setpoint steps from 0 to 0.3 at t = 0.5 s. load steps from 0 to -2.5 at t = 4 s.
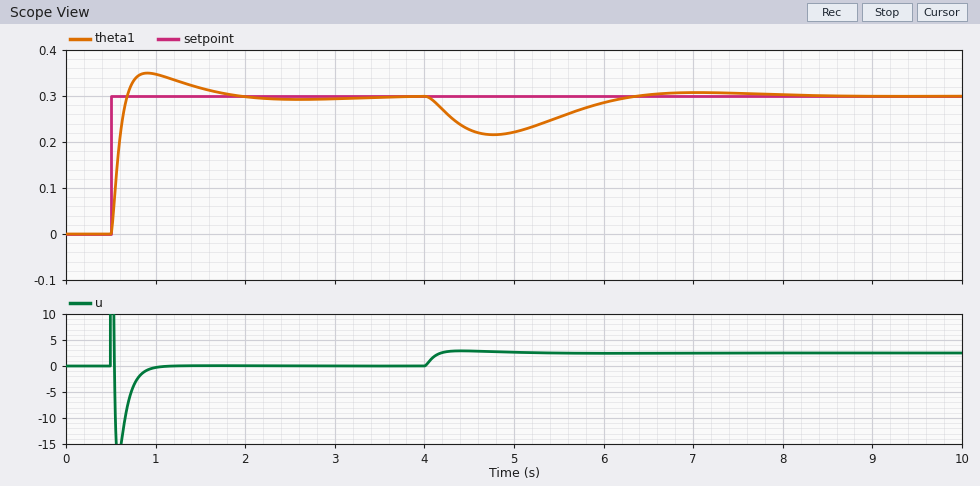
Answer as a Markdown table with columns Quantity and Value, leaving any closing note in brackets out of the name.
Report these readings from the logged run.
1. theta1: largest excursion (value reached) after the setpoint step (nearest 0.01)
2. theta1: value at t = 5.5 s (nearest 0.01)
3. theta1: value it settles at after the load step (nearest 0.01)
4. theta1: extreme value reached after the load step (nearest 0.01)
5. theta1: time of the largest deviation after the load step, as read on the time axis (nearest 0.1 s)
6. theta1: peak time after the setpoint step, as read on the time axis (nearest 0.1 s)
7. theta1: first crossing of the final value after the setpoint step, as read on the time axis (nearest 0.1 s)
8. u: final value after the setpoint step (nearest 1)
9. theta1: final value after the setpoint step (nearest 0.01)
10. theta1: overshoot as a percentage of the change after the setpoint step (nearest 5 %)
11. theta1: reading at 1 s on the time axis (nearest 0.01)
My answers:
| Quantity | Value |
|---|---|
| theta1: largest excursion (value reached) after the setpoint step | 0.35 |
| theta1: value at t = 5.5 s | 0.25 |
| theta1: value it settles at after the load step | 0.30 |
| theta1: extreme value reached after the load step | 0.22 |
| theta1: time of the largest deviation after the load step, as read on the time axis | 4.8 s |
| theta1: peak time after the setpoint step, as read on the time axis | 0.9 s |
| theta1: first crossing of the final value after the setpoint step, as read on the time axis | 0.7 s |
| u: final value after the setpoint step | 0 |
| theta1: final value after the setpoint step | 0.30 |
| theta1: overshoot as a percentage of the change after the setpoint step | 15 % |
| theta1: reading at 1 s on the time axis | 0.35 |
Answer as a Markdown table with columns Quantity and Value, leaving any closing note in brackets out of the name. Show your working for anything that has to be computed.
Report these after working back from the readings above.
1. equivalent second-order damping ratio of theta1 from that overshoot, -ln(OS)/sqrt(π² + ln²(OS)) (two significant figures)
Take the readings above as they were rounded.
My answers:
| Quantity | Value |
|---|---|
| equivalent second-order damping ratio of theta1 from that overshoot, -ln(OS)/sqrt(π² + ln²(OS)) | ln(0.15) = -1.897; 1.897 / sqrt(9.870 + 3.599) = 0.52 |
